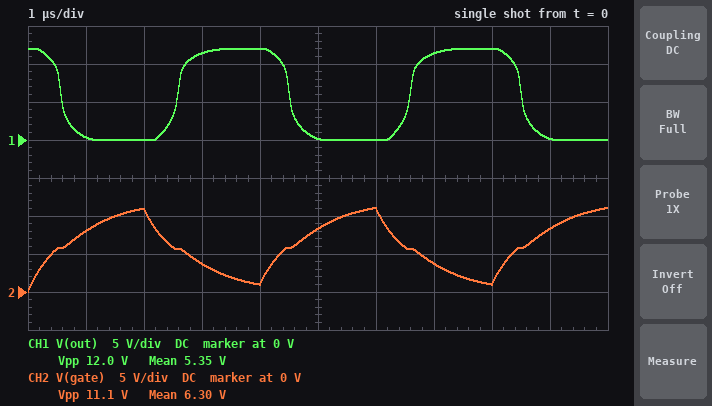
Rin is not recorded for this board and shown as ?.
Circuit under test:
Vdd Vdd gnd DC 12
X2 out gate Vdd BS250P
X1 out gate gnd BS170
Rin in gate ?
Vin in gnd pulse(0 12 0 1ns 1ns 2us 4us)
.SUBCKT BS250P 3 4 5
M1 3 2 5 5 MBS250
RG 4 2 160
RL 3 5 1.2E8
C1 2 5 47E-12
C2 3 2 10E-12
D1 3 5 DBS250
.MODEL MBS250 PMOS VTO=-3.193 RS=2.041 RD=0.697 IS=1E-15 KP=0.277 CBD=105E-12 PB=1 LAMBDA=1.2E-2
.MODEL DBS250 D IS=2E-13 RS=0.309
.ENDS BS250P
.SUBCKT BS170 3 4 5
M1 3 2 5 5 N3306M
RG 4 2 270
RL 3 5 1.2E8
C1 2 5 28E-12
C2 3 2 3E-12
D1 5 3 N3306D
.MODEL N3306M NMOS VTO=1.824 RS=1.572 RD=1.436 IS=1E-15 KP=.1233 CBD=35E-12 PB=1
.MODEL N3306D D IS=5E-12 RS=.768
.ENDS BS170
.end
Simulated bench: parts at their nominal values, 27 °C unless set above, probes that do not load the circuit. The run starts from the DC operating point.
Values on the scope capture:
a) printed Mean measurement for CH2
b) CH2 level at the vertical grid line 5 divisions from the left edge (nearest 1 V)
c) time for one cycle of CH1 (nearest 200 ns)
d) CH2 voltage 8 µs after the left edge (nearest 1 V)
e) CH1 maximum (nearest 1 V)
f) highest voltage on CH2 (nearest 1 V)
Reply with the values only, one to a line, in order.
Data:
6.30 V
8 V
4.0 µs
1 V
12 V
11 V
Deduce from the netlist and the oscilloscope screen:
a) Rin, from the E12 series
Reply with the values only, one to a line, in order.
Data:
8.2 kΩ
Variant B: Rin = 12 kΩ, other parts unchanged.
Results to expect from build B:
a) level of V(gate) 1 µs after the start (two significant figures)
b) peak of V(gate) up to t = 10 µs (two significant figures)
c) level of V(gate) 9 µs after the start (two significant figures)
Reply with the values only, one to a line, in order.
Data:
6.2 V
10 V
7.1 V
